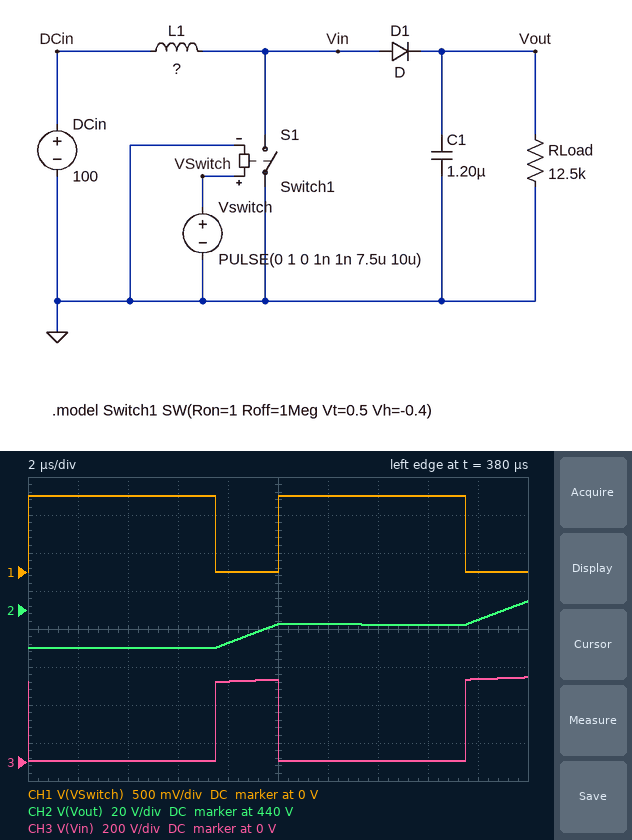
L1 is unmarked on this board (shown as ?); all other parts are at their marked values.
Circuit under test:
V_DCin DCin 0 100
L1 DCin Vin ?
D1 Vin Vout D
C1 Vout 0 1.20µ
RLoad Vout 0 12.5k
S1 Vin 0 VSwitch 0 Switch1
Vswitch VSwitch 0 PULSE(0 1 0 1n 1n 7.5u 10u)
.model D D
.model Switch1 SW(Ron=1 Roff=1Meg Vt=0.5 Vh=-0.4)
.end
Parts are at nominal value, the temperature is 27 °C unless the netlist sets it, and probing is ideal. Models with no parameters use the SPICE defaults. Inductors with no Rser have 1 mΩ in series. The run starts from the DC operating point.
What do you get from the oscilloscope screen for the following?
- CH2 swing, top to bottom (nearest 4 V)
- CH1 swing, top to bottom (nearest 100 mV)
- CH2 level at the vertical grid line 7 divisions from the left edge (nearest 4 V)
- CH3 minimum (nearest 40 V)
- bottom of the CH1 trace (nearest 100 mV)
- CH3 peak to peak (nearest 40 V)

24 V
1.0 V
432 V
0 V
0 V
440 V
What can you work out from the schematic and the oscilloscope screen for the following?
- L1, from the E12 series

2.7 mH
